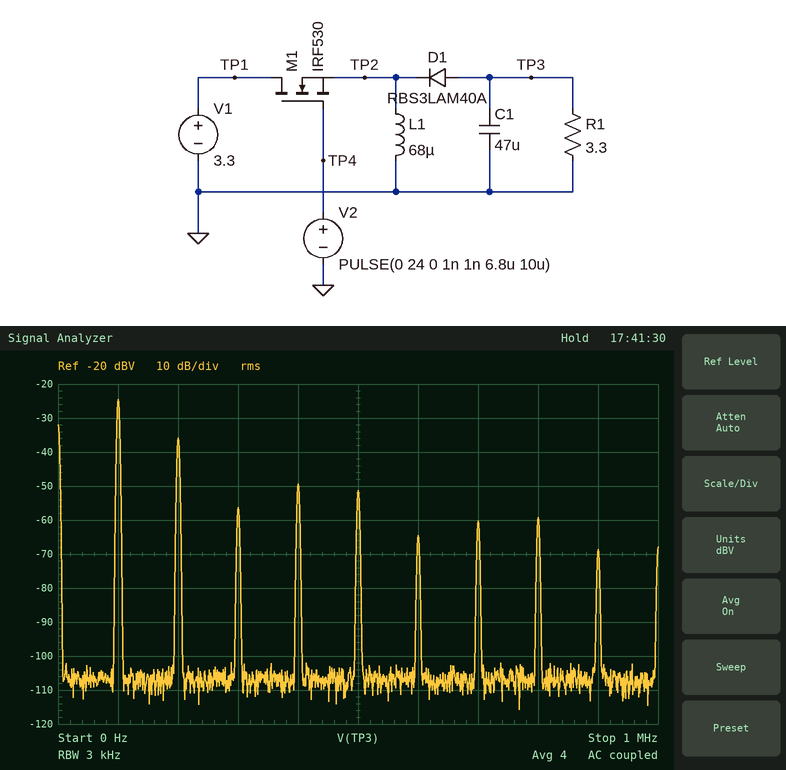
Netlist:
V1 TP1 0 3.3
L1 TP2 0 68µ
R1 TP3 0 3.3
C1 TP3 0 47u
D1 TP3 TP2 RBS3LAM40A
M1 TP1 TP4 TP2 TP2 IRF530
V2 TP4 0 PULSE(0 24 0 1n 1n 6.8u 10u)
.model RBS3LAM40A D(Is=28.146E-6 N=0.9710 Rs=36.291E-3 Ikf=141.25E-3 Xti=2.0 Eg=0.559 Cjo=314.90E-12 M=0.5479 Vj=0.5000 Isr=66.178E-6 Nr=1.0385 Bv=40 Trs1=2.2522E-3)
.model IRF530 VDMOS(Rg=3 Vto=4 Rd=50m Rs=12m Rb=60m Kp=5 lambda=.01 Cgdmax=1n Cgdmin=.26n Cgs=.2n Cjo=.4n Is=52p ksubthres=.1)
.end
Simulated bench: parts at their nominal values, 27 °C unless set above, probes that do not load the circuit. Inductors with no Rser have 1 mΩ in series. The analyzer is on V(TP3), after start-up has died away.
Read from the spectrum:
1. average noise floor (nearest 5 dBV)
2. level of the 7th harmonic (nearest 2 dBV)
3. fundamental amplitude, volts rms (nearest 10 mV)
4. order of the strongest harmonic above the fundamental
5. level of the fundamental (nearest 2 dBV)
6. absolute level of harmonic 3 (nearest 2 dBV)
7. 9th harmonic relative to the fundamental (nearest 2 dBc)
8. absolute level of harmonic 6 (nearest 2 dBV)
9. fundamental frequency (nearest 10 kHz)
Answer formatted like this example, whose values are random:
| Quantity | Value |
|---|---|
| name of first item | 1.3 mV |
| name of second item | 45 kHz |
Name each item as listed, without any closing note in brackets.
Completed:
| Quantity | Value |
|---|---|
| average noise floor | -105 dBV |
| level of the 7th harmonic | -60 dBV |
| fundamental amplitude, volts rms | 60 mV |
| order of the strongest harmonic above the fundamental | 2 |
| level of the fundamental | -24 dBV |
| absolute level of harmonic 3 | -56 dBV |
| 9th harmonic relative to the fundamental | -44 dBc |
| absolute level of harmonic 6 | -64 dBV |
| fundamental frequency | 100 kHz |
